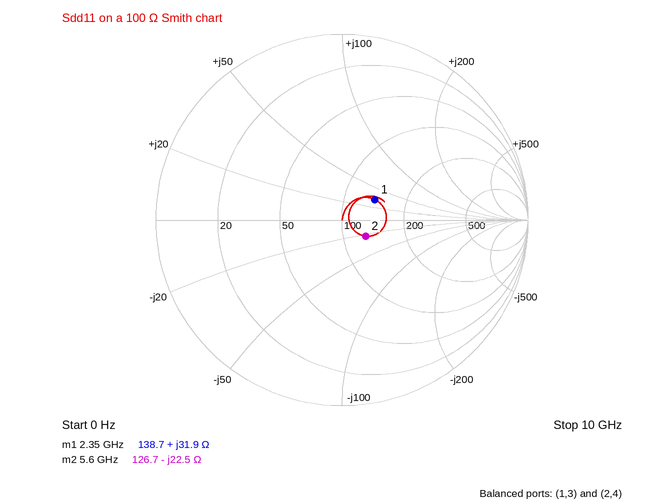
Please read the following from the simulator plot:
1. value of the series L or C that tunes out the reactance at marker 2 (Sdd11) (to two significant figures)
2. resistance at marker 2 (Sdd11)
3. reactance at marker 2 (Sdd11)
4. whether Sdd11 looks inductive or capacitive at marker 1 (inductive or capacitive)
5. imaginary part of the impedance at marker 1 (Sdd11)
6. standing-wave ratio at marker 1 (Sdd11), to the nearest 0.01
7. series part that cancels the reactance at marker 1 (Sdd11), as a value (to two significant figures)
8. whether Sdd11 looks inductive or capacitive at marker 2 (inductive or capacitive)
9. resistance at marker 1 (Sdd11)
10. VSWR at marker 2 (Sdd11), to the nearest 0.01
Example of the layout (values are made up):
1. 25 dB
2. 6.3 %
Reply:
1. 640 pH
2. 126.7 Ω
3. -22.5 Ω
4. inductive
5. +31.9 Ω
6. 1.53
7. 2.1 pF
8. capacitive
9. 138.7 Ω
10. 1.36
